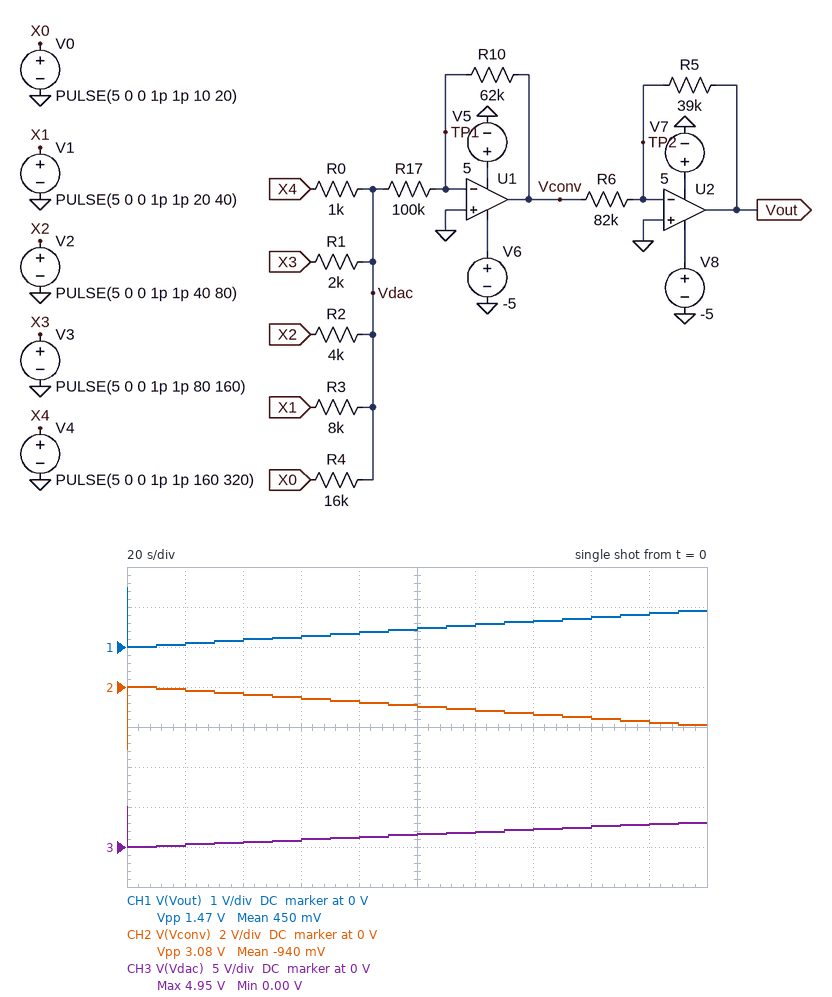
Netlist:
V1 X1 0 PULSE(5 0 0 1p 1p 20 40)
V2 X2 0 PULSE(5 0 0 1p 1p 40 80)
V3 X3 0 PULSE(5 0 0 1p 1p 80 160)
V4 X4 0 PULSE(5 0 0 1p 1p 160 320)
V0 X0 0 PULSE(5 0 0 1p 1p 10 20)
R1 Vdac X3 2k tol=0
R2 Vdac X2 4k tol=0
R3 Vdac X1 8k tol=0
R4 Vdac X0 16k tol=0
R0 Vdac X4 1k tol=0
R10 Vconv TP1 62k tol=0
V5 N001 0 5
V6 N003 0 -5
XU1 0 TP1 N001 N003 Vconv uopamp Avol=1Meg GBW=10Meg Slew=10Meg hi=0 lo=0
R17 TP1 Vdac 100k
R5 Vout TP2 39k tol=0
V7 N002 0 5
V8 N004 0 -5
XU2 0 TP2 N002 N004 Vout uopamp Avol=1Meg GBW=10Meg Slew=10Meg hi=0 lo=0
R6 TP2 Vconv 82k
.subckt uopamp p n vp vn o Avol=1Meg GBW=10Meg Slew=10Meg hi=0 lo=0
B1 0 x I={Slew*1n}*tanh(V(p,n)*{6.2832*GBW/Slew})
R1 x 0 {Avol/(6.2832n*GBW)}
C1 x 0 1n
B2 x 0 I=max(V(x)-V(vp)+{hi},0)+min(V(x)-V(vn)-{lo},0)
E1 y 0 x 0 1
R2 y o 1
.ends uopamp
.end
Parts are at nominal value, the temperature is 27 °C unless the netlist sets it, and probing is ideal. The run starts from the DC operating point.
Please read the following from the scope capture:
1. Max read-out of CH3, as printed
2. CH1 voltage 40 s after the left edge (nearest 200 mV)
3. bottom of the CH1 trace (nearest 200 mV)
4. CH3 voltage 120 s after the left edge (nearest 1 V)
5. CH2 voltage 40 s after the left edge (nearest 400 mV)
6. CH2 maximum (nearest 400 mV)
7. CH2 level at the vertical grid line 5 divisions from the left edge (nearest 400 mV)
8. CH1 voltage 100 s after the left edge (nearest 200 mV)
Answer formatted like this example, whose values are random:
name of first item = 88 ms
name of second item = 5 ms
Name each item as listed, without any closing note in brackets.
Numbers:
Max read-out of CH3, as printed = 4.95 V
CH1 voltage 40 s after the left edge = 200 mV
bottom of the CH1 trace = 0 V
CH3 voltage 120 s after the left edge = 2 V
CH2 voltage 40 s after the left edge = -400 mV
CH2 maximum = 0 V
CH2 level at the vertical grid line 5 divisions from the left edge = -800 mV
CH1 voltage 100 s after the left edge = 400 mV
